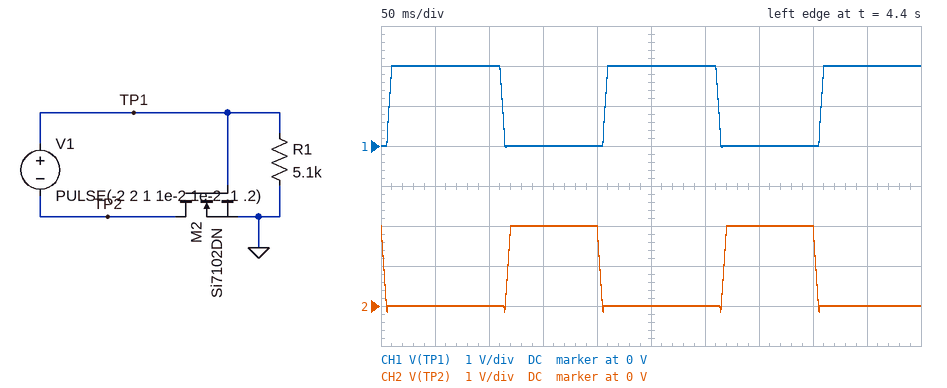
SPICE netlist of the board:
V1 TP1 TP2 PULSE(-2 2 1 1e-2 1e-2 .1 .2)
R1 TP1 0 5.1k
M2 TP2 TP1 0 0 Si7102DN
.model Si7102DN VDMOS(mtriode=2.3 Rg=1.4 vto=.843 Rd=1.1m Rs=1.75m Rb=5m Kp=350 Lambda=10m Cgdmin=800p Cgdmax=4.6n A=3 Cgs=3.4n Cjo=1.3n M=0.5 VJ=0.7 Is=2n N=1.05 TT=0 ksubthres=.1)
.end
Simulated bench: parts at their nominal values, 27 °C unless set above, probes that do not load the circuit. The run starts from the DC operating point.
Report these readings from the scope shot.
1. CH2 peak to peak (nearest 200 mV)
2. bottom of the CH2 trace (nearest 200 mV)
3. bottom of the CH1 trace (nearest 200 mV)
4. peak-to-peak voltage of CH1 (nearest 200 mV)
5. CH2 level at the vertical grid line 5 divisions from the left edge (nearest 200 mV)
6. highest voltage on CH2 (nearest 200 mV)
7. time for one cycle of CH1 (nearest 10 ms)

2.2 V
-200 mV
0 V
2.0 V
0 V
2.0 V
200 ms
